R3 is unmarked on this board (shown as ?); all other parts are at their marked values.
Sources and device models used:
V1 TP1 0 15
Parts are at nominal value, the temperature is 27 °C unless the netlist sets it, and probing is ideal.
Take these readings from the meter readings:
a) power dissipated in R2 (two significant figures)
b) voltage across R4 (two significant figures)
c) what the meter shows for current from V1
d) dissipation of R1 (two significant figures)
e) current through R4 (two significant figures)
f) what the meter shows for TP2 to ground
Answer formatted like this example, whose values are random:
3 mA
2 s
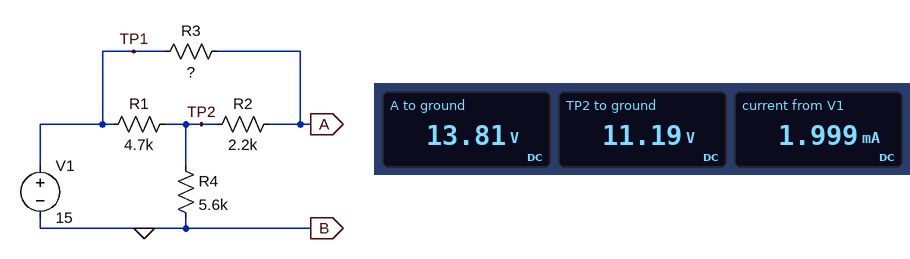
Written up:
3.1 mW
11 V
1.999 mA
3.1 mW
2.0 mA
11.19 V
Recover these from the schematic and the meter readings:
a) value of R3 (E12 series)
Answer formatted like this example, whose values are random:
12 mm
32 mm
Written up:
1 kΩ
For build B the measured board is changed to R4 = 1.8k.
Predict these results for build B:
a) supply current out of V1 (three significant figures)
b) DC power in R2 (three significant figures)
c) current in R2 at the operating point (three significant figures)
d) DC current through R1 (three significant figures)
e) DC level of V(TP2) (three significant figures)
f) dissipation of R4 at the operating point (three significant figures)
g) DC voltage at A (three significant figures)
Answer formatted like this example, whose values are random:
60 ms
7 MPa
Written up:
4.05 mA
12.8 mW
2.41 mA
1.64 mA
7.29 V
29.5 mW
12.6 V
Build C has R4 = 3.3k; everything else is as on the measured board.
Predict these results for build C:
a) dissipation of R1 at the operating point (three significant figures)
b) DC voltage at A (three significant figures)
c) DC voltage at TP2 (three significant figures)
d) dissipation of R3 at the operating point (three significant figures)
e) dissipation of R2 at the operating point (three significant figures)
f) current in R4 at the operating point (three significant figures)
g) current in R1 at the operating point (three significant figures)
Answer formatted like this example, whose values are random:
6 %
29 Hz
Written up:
6.41 mW
13.3 V
9.51 V
2.94 mW
6.47 mW
2.88 mA
1.17 mA
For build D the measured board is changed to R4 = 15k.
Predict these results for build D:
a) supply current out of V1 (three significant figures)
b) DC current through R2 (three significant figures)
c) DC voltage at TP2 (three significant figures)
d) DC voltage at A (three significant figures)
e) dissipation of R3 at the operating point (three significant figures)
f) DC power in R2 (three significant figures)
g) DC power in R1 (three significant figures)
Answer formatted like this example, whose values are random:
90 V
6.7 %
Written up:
887 µA
528 µA
13.3 V
14.5 V
279 µW
613 µW
607 µW
